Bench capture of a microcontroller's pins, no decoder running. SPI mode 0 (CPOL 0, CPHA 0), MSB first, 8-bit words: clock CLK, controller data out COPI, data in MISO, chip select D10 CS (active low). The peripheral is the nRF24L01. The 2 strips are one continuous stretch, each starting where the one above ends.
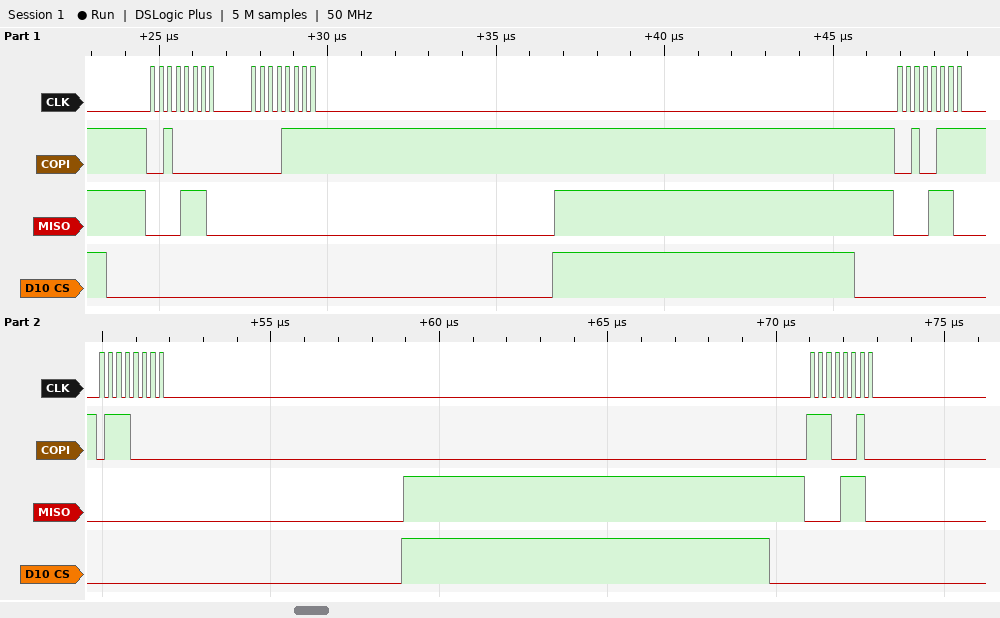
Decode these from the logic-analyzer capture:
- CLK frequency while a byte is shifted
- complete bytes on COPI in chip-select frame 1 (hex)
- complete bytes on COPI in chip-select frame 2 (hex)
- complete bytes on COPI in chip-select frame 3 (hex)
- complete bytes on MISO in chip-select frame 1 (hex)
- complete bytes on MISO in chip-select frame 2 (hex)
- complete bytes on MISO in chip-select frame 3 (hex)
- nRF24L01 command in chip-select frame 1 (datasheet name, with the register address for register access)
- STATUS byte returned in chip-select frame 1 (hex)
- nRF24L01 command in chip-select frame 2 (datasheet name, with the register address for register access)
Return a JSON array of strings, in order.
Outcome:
["4 MHz", "20 0F", "27 70", "E2", "0E 00", "0E 00", "0E", "W_REGISTER 0x00", "0x0E", "W_REGISTER 0x07"]
